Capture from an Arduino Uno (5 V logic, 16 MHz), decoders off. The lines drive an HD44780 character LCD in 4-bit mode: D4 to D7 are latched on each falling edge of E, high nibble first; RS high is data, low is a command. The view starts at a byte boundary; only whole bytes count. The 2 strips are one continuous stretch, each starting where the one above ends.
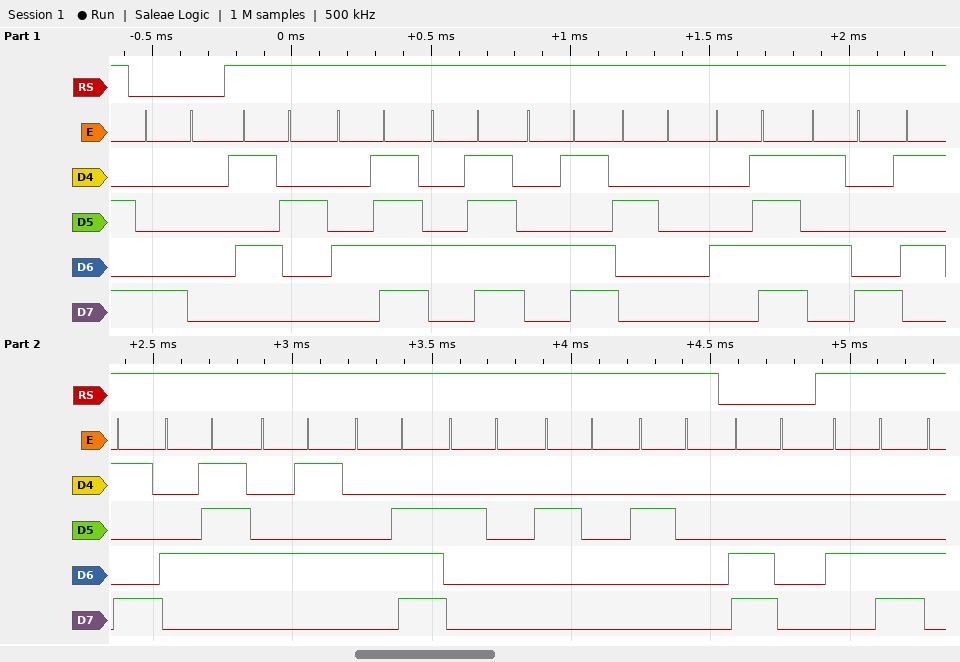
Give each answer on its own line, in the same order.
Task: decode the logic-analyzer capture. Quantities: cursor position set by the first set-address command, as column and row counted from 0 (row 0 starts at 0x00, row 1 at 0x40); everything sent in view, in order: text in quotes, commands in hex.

column 0, row 0
0x80 "ROOM OXYGEN   " 0xC0 "L"
